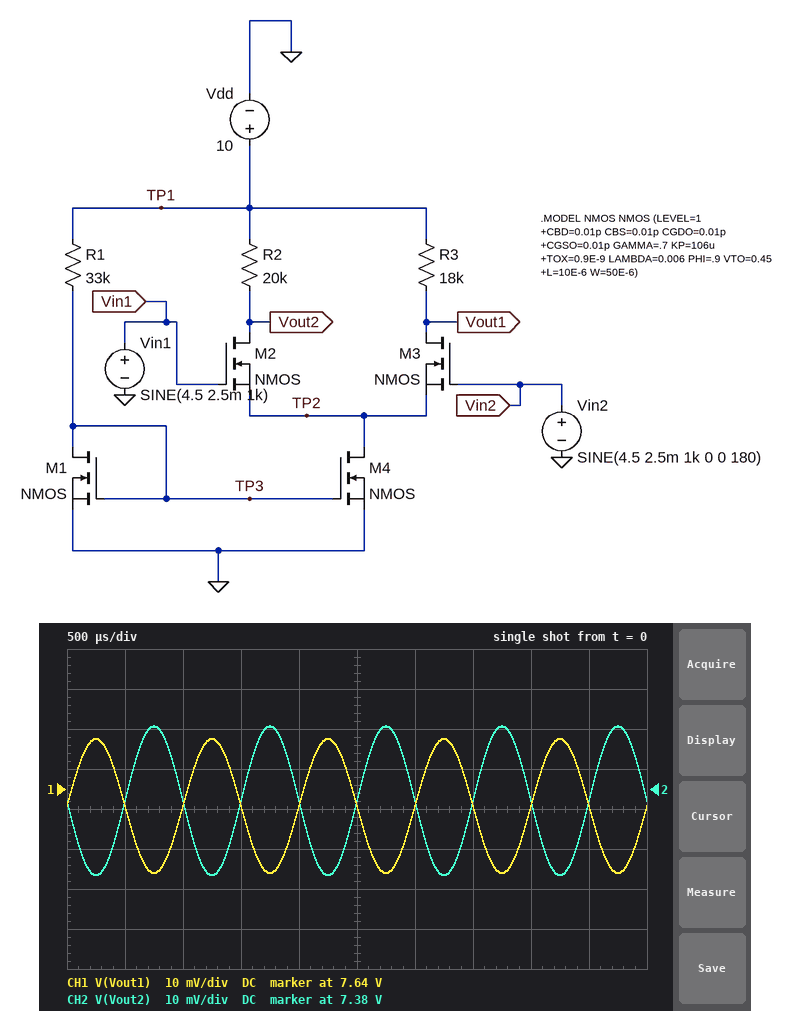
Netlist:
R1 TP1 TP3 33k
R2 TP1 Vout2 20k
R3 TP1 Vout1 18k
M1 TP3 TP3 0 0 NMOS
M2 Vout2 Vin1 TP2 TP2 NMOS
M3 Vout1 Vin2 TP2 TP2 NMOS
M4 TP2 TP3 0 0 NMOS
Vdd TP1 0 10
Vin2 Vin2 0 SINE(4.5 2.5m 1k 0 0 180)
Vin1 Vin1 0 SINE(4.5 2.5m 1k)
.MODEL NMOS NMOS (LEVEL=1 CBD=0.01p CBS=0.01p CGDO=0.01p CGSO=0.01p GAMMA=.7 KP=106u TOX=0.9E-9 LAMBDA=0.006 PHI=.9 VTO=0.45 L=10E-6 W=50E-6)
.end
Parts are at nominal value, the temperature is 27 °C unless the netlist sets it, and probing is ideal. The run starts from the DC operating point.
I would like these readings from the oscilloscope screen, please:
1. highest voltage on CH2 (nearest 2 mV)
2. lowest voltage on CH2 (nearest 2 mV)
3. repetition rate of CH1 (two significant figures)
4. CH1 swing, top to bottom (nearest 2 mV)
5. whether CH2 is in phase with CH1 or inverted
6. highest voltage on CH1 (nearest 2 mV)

7.396 V
7.358 V
1.0 kHz
34 mV
inverted
7.652 V
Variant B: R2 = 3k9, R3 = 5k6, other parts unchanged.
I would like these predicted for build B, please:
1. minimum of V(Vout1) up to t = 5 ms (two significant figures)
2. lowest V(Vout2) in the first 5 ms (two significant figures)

9.3 V
9.5 V
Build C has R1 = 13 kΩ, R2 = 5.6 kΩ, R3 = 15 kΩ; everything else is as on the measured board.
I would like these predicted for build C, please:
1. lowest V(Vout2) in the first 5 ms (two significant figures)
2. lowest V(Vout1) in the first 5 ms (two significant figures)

8.2 V
5.4 V
